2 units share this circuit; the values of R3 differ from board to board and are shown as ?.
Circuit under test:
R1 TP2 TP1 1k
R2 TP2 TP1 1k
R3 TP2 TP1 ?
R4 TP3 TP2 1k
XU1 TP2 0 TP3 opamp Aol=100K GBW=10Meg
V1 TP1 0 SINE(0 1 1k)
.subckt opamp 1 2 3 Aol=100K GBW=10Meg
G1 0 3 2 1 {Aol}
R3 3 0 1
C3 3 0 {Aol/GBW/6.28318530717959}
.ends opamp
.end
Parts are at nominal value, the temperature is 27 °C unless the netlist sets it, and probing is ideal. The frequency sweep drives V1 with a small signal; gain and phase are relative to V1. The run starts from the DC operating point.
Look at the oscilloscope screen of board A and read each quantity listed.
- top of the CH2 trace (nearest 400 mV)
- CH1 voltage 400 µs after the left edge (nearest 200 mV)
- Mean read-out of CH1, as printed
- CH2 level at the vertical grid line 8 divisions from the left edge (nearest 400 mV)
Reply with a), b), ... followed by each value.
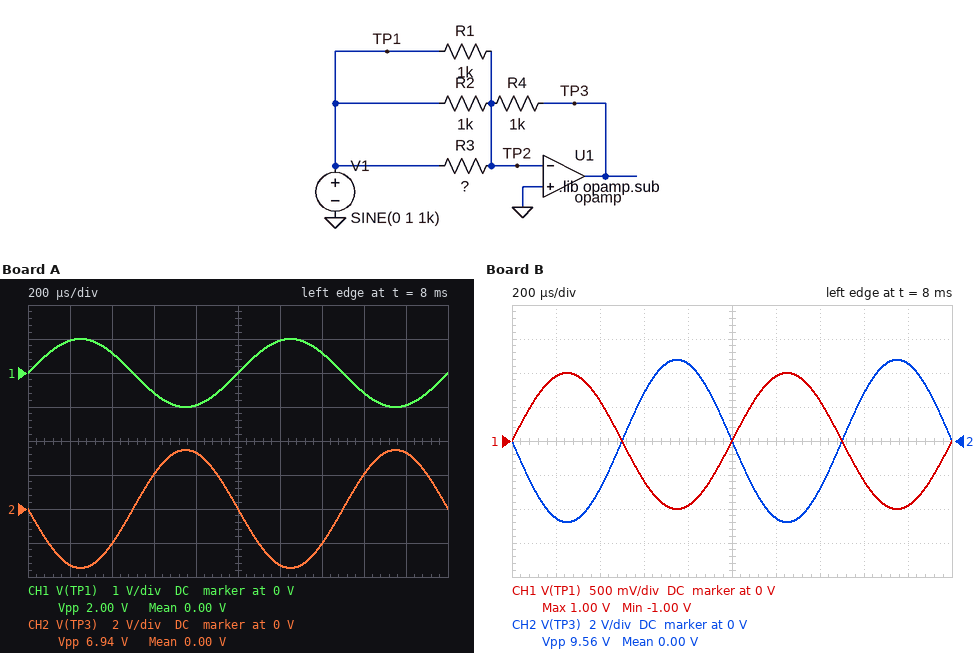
a) 3.6 V
b) 600 mV
c) 0.00 V
d) 2.0 V
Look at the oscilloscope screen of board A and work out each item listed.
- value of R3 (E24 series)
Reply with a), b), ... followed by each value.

a) 680 Ω
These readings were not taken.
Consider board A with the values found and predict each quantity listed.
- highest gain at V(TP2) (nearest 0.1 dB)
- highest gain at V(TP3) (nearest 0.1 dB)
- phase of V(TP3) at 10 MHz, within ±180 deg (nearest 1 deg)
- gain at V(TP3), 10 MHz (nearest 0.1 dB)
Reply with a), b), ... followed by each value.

a) -2.2 dB
b) 10.8 dB
c) 103 deg
d) -2.4 dB
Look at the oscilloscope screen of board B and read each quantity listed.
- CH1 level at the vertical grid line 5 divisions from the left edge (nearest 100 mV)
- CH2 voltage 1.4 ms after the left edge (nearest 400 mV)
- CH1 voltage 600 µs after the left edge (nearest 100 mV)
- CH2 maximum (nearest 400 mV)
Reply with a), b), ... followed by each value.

a) 0 V
b) -2.8 V
c) -600 mV
d) 4.8 V
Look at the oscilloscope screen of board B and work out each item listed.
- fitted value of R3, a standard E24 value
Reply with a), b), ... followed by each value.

a) 360 Ω
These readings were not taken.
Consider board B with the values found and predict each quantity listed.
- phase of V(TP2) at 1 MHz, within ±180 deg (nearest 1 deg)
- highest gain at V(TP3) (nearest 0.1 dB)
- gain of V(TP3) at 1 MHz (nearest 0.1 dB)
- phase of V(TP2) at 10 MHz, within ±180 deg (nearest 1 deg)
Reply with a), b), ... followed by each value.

a) 60 deg
b) 13.6 dB
c) 12.3 dB
d) 10 deg
